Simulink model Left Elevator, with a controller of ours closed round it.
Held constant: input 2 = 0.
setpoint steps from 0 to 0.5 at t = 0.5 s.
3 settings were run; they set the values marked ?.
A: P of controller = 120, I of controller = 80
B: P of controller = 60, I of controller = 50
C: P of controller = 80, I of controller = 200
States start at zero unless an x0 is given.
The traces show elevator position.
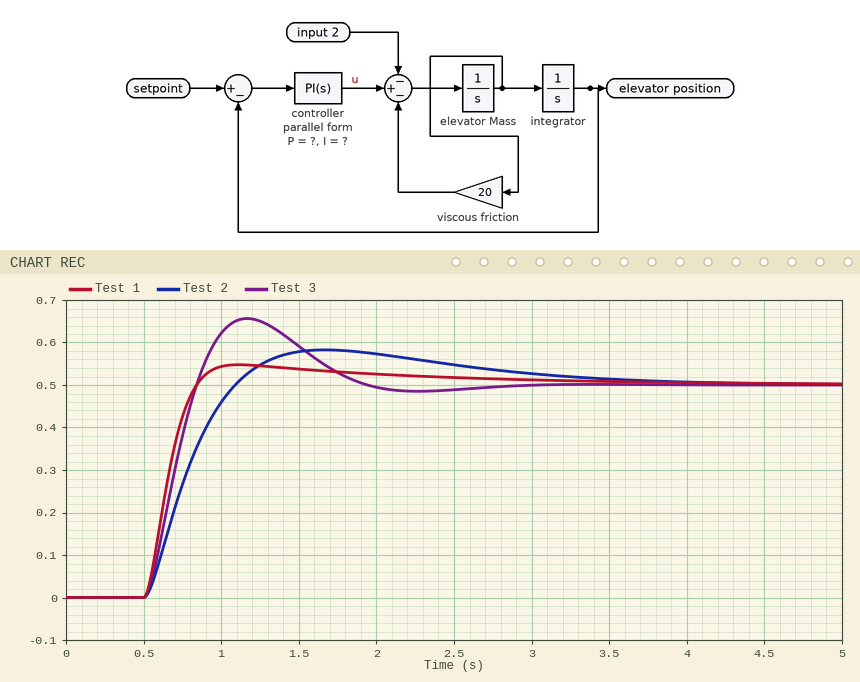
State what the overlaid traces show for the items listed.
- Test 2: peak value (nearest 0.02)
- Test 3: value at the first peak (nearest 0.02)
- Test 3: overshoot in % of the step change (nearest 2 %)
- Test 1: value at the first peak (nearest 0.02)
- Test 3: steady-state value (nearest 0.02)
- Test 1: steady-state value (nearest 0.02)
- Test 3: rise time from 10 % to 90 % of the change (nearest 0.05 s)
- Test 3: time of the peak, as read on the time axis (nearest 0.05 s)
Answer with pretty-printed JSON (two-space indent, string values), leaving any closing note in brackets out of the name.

{
  "Test 2: peak value": "0.58",
  "Test 3: value at the first peak": "0.66",
  "Test 3: overshoot in % of the step change": "32 %",
  "Test 1: value at the first peak": "0.54",
  "Test 3: steady-state value": "0.50",
  "Test 1: steady-state value": "0.50",
  "Test 3: rise time from 10 % to 90 % of the change": "0.25 s",
  "Test 3: time of the peak, as read on the time axis": "1.15 s"
}
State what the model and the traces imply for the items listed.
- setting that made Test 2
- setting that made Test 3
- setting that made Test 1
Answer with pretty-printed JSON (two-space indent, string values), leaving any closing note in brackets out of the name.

{
  "setting that made Test 2": "B",
  "setting that made Test 3": "C",
  "setting that made Test 1": "A"
}
